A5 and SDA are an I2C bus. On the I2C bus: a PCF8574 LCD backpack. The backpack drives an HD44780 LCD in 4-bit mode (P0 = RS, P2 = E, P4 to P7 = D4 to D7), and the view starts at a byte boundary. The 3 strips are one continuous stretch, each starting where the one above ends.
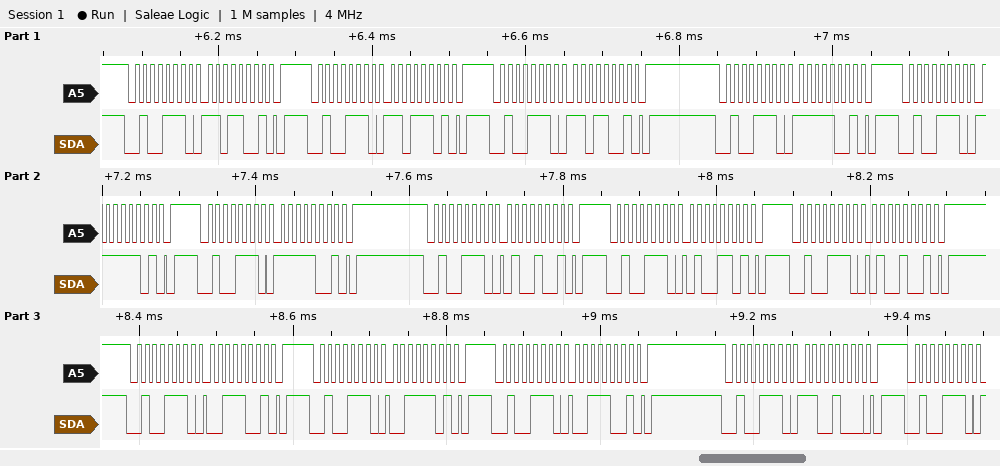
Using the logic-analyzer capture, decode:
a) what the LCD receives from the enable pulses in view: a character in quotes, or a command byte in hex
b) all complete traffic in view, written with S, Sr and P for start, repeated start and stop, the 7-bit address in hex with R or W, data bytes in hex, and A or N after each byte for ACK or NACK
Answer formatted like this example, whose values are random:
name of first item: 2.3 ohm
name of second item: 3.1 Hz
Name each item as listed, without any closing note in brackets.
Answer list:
what the LCD receives from the enable pulses in view: a character in quotes, or a command byte in hex: data 0xDF 'C'
all complete traffic in view, written with S, Sr and P for start, repeated start and stop, the 7-bit address in hex with R or W, data bytes in hex, and A or N after each byte for ACK or NACK: S 27W A D9 A P S 27W A DD A P S 27W A D9 A P S 27W A F9 A P S 27W A FD A P S 27W A F9 A P S 27W A 49 A P S 27W A 4D A P S 27W A 49 A P S 27W A 39 A P S 27W A 3D A P S 27W A 39 A P S 27W A C8 A P S 27W A
